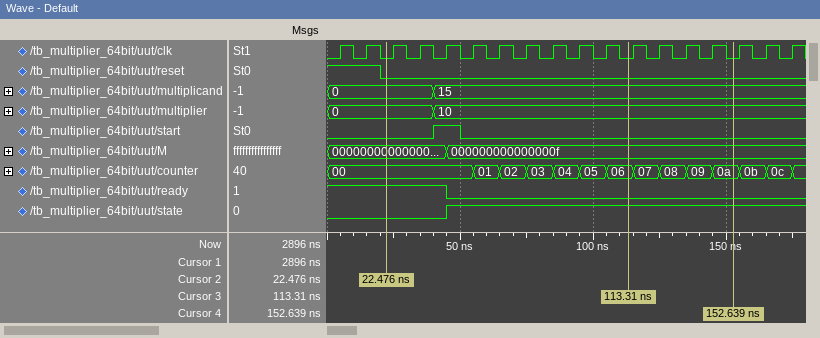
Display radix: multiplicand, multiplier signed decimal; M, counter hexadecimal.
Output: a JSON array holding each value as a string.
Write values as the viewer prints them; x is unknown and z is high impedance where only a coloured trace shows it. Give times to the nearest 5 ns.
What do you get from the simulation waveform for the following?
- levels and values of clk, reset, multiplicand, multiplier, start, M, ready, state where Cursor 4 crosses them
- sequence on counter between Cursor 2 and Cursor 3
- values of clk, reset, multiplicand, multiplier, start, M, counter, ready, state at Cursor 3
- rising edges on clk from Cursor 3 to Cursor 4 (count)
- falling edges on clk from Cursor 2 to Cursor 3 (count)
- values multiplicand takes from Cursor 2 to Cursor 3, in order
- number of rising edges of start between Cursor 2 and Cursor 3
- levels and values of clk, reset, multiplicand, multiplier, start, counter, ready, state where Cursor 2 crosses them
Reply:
["clk=0, reset=0, multiplicand=15, multiplier=10, start=0, M=000000000000000f, ready=0, state=1", "00, 01, 02, 03, 04, 05, 06", "clk=0, reset=0, multiplicand=15, multiplier=10, start=0, M=000000000000000f, counter=06, ready=0, state=1", "4", "9", "0, 15", "1", "clk=0, reset=0, multiplicand=0, multiplier=0, start=0, counter=00, ready=1, state=0"]
